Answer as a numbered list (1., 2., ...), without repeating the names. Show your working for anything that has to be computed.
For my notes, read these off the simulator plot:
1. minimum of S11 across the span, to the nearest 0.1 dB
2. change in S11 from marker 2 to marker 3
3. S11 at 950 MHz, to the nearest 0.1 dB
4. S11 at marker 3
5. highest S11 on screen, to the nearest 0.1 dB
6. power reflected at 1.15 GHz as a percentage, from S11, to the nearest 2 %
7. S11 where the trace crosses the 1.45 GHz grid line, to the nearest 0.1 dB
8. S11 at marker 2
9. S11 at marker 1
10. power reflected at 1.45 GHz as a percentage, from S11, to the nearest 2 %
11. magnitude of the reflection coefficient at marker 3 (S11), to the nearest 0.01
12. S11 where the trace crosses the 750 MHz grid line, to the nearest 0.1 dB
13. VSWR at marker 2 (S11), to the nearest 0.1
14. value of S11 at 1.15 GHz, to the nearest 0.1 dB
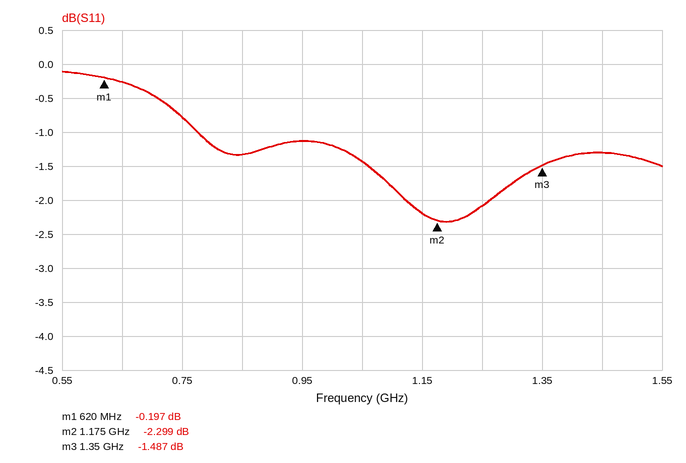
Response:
1. -2.3 dB
2. -1.487 − (-2.299) = 0.812 dB
3. -1.1 dB
4. -1.487 dB
5. -0.1 dB
6. 10^(-2.2/10) ≈ 60 %
7. -1.3 dB
8. -2.299 dB
9. -0.197 dB
10. 10^(-1.3/10) ≈ 74 %
11. 10^(-1.487/20) ≈ 0.84
12. -0.8 dB
13. (1 + 0.7674)/(1 − 0.7674) ≈ 7.6
14. -2.2 dB
